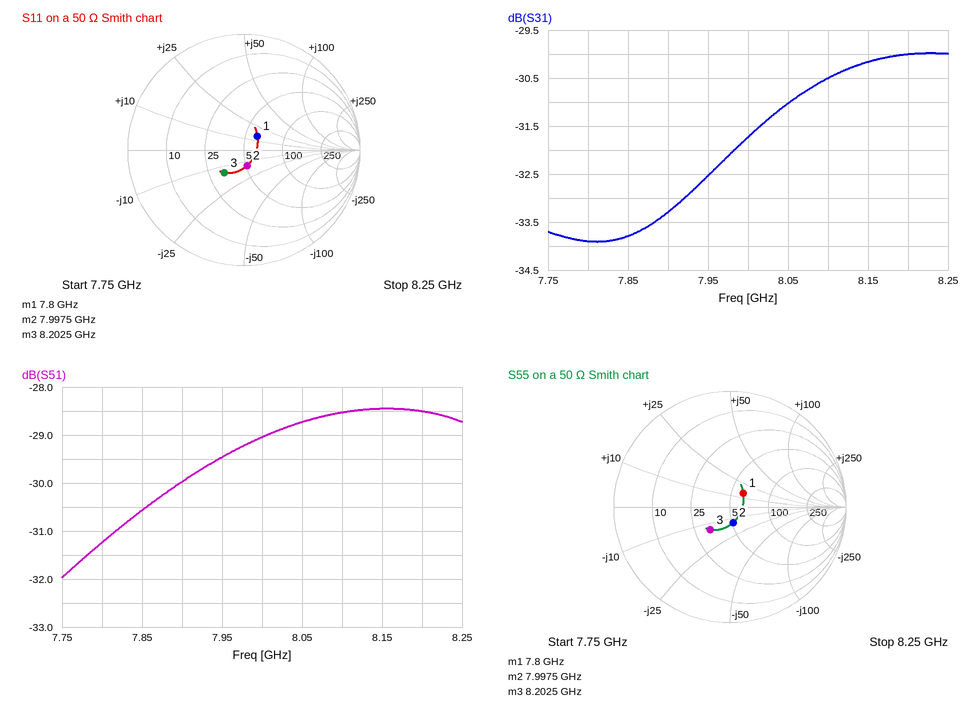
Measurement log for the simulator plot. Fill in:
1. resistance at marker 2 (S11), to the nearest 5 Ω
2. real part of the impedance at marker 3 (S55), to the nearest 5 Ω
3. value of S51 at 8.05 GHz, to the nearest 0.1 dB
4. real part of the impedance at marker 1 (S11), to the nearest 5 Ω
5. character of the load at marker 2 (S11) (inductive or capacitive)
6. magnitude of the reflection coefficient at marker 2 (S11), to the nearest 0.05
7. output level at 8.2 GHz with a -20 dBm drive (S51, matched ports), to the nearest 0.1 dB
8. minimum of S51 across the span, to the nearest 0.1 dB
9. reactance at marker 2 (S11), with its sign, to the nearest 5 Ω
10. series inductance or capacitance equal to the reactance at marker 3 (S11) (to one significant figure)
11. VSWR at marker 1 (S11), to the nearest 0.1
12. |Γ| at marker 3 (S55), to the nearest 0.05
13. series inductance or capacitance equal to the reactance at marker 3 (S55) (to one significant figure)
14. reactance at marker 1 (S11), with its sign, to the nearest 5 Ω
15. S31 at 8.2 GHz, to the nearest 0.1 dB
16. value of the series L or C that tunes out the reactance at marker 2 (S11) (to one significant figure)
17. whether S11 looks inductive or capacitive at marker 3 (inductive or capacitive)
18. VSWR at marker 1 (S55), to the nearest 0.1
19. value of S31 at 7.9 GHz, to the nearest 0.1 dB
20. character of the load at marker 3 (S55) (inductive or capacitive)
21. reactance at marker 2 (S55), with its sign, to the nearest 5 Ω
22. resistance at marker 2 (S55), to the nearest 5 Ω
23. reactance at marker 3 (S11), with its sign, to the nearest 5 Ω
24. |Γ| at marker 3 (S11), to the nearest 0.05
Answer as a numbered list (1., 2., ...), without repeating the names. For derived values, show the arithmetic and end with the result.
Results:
1. 50 Ω
2. 35 Ω
3. -28.7 dB
4. 60 Ω
5. capacitive
6. 0.15
7. -20 dBm + (-28.5 dB) = -48.5 dBm
8. -32.0 dB
9. -15 Ω
10. C = 1/(2π × 8.2025 GHz × 15 Ω) ≈ 1 pF
11. 1.4
12. 0.25
13. C = 1/(2π × 8.2025 GHz × 15 Ω) ≈ 1 pF
14. +15 Ω
15. -30.0 dB
16. L = 15 Ω/(2π × 7.9975 GHz) ≈ 299 pH, so 300 pH to one significant figure
17. capacitive
18. 1.4
19. -33.3 dB
20. capacitive
21. -15 Ω
22. 50 Ω
23. -15 Ω
24. 0.25
